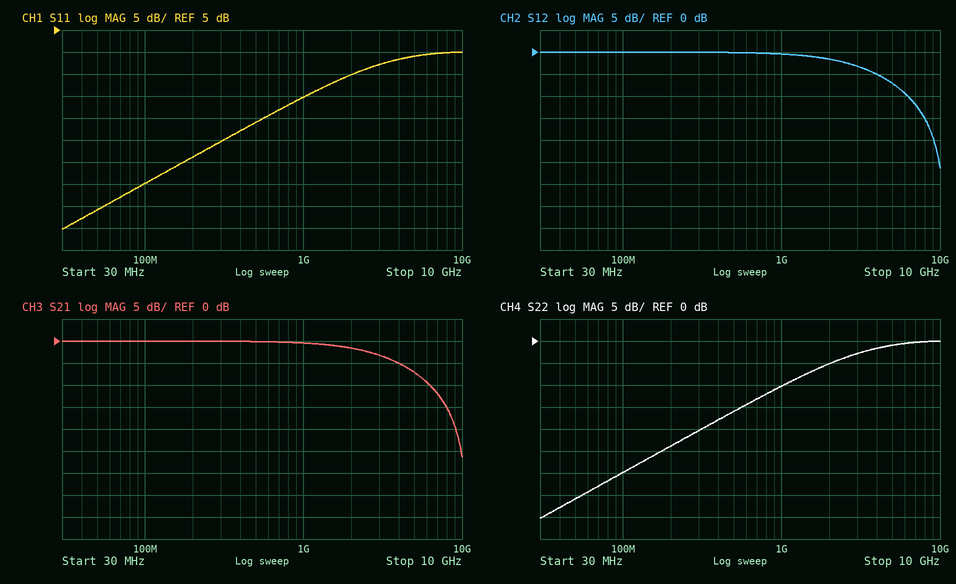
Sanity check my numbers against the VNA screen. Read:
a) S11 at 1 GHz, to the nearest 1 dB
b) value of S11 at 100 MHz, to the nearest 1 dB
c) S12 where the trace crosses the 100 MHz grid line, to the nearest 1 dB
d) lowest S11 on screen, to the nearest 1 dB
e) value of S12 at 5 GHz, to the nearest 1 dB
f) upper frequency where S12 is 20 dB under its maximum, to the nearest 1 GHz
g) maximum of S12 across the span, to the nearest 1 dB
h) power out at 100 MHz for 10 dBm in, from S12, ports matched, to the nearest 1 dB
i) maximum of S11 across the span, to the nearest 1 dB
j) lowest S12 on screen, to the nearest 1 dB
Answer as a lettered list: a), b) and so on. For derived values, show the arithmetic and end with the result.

a) -10 dB
b) -30 dB
c) 0 dB
d) -40 dB
e) -7 dB
f) 9 GHz
g) 0 dB
h) 10 dBm + (0 dB) = 10 dBm
i) 0 dB
j) -26 dB
